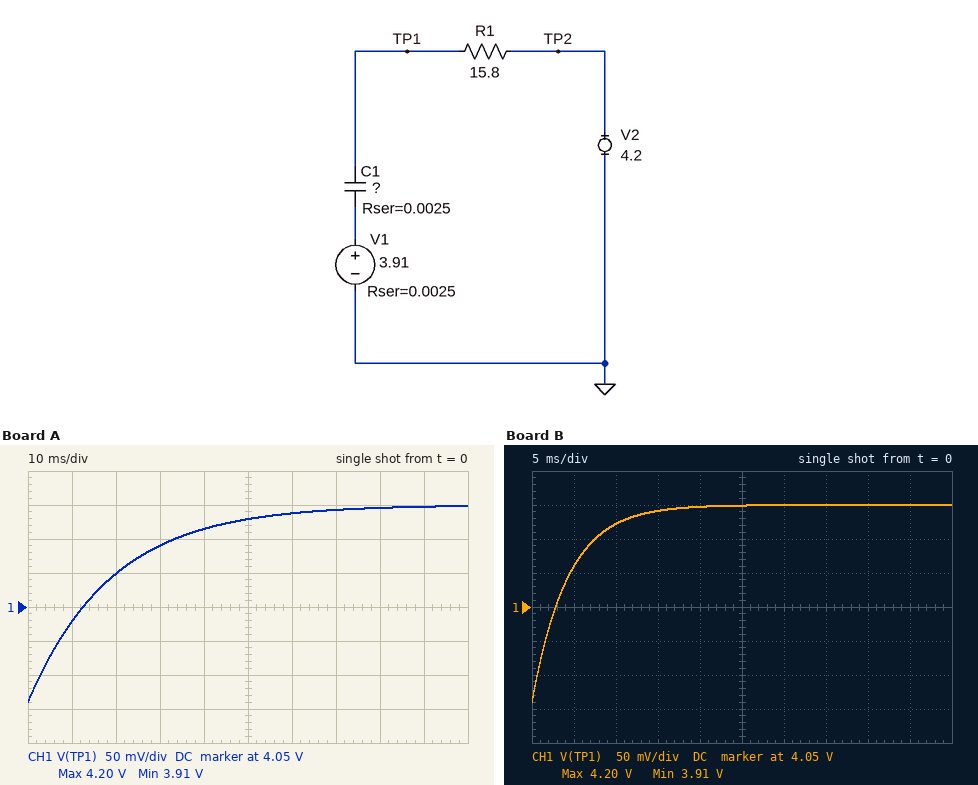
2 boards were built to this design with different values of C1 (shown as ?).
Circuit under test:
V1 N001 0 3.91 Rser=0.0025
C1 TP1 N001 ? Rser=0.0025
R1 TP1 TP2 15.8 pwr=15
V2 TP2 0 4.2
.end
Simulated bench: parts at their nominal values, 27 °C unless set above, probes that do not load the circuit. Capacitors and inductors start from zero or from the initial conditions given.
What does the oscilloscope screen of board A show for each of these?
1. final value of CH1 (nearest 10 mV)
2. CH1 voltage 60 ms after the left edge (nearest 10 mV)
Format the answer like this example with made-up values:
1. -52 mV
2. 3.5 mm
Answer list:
1. 4.20 V
2. 4.19 V
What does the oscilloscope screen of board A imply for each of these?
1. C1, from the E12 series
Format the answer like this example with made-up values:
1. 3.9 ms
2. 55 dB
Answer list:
1. 1.2 mF
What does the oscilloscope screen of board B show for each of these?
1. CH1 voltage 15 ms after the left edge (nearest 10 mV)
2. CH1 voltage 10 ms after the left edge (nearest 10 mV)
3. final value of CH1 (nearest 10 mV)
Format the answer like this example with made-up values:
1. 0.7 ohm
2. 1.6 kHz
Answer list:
1. 4.19 V
2. 4.17 V
3. 4.20 V
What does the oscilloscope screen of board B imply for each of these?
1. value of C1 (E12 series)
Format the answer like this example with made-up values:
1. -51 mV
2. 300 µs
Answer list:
1. 270 µF
